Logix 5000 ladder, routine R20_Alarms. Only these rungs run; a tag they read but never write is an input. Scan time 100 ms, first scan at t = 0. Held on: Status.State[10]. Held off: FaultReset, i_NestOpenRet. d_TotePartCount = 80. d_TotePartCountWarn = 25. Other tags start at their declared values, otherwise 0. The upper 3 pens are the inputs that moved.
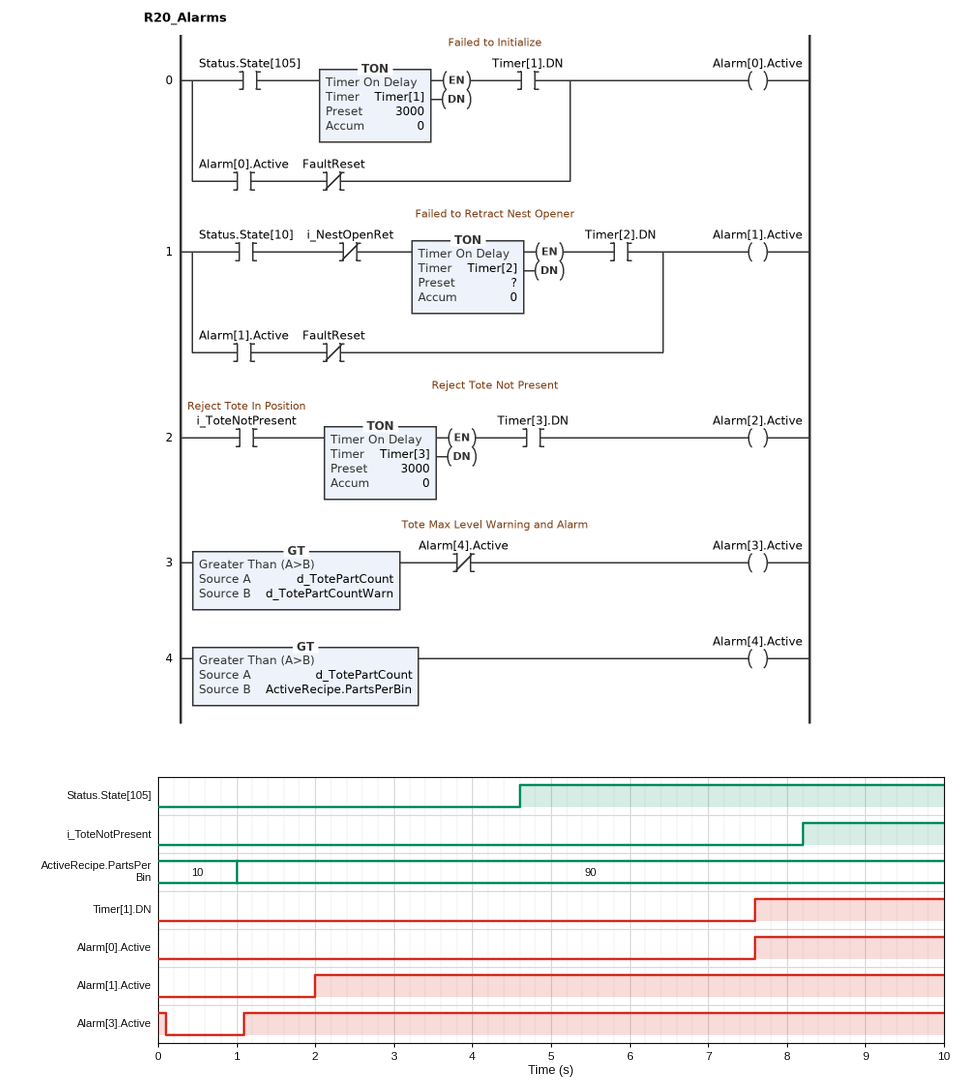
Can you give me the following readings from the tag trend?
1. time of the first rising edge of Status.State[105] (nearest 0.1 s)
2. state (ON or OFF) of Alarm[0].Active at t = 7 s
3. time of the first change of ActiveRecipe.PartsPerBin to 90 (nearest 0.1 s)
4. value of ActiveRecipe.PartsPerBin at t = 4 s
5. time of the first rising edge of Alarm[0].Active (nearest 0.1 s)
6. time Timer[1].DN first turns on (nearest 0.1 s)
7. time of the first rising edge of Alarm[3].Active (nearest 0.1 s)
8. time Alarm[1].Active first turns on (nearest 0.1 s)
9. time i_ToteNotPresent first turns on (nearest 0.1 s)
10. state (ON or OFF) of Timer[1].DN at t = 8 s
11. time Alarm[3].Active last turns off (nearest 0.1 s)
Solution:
4.6 s
OFF
1.0 s
90
7.6 s
7.6 s
1.1 s
2.0 s
8.2 s
ON
0.1 s
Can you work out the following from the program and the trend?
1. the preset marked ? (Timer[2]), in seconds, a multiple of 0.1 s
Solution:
2.0 s
